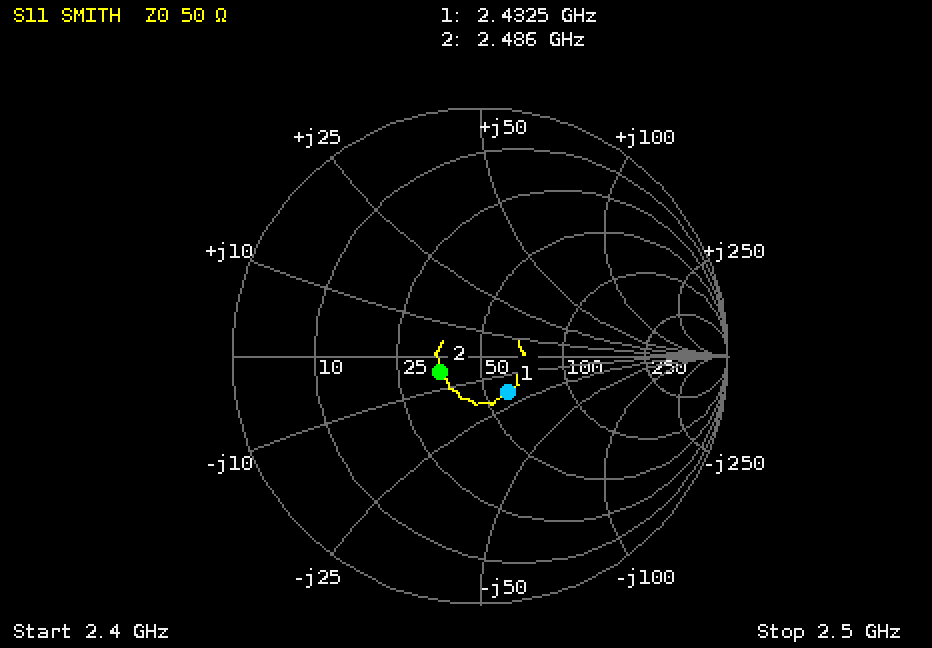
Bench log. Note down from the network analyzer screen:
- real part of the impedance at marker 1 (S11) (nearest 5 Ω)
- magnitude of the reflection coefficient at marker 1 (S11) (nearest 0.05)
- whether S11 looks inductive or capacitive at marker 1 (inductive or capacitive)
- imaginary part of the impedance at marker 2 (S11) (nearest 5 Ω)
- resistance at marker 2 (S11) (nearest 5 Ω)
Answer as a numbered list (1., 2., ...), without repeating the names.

1. 60 Ω
2. 0.20
3. capacitive
4. -5 Ω
5. 35 Ω
